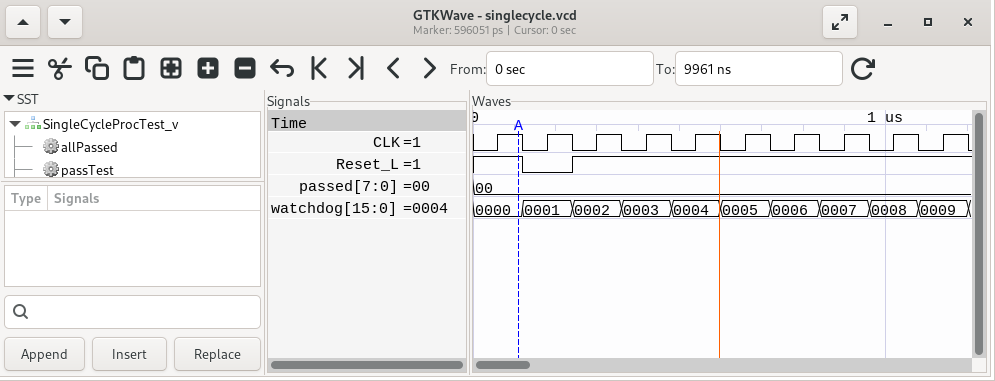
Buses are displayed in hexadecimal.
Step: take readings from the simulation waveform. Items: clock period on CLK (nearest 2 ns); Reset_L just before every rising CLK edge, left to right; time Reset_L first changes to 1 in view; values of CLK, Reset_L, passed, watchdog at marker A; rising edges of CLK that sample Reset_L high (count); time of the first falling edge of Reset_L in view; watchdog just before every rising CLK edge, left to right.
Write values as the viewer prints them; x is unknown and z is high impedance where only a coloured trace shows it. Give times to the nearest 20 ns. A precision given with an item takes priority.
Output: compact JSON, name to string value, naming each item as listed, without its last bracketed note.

{"clock period on CLK": "120 ns", "Reset_L just before every rising CLK edge, left to right": "1 0 1 1 1 1 1 1 1 1", "time Reset_L first changes to 1 in view": "240 ns", "values of CLK, Reset_L, passed, watchdog at marker A": "CLK=1, Reset_L=1, passed=00, watchdog=0000", "rising edges of CLK that sample Reset_L high": "9", "time of the first falling edge of Reset_L in view": "120 ns", "watchdog just before every rising CLK edge, left to right": "0000, 0001, 0002, 0003, 0004, 0005, 0006, 0007, 0008, 0009"}
